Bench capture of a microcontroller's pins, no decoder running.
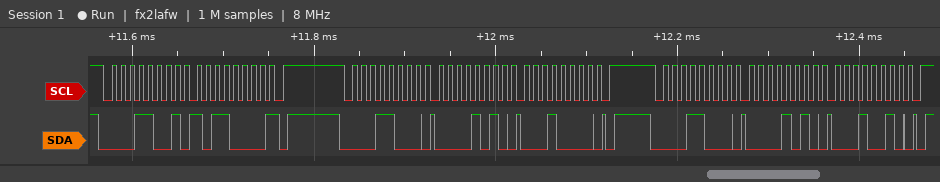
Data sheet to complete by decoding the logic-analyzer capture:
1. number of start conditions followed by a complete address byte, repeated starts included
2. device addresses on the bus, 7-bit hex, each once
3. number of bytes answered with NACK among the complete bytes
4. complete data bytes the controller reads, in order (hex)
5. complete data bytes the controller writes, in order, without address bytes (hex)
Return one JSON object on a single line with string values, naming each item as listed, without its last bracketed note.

{"number of start conditions followed by a complete address byte, repeated starts included": "3", "device addresses on the bus, 7-bit hex, each once": "0x0C", "number of bytes answered with NACK among the complete bytes": "1", "complete data bytes the controller reads, in order": "B0", "complete data bytes the controller writes, in order, without address bytes": "0A 10 0A 12"}
